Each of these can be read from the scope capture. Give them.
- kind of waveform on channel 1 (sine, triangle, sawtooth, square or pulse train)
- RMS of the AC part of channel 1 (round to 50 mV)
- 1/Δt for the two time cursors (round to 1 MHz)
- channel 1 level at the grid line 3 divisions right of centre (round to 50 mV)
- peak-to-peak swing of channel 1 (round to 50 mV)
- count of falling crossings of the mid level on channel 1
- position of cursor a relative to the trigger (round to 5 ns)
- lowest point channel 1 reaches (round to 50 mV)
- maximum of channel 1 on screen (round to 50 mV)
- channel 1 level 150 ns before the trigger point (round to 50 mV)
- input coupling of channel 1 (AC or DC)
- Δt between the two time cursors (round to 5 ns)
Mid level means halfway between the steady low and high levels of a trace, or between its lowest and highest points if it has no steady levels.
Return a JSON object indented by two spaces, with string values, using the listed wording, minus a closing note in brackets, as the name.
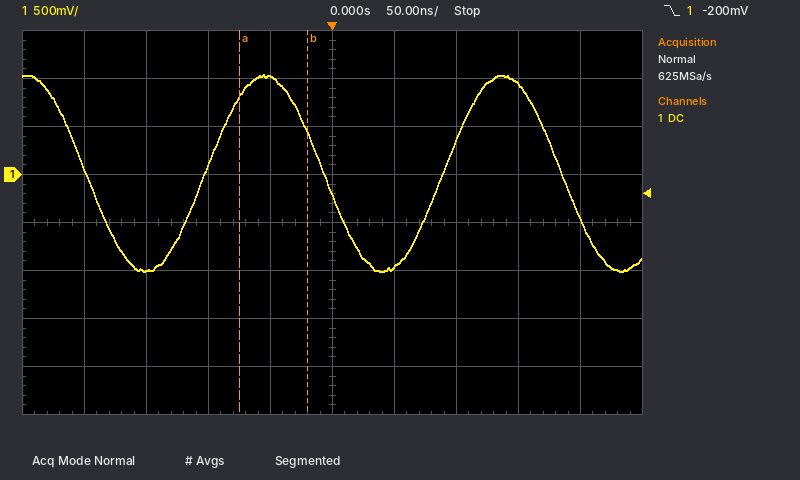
{
  "kind of waveform on channel 1": "sine",
  "RMS of the AC part of channel 1": "700 mV",
  "1/Δt for the two time cursors": "18 MHz",
  "channel 1 level at the grid line 3 divisions right of centre": "950 mV",
  "peak-to-peak swing of channel 1": "2.05 V",
  "count of falling crossings of the mid level on channel 1": "3",
  "position of cursor a relative to the trigger": "-75 ns",
  "lowest point channel 1 reaches": "-1.00 V",
  "maximum of channel 1 on screen": "1.05 V",
  "channel 1 level 150 ns before the trigger point": "-1.00 V",
  "input coupling of channel 1": "DC",
  "Δt between the two time cursors": "55 ns"
}
